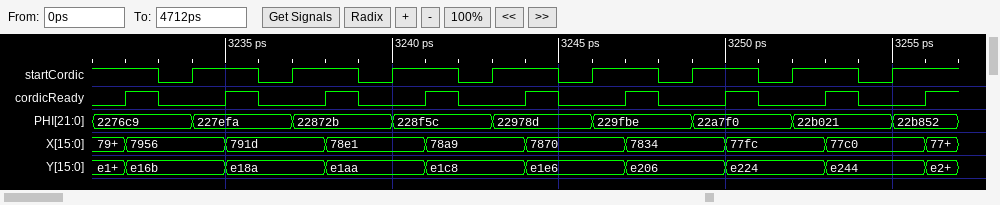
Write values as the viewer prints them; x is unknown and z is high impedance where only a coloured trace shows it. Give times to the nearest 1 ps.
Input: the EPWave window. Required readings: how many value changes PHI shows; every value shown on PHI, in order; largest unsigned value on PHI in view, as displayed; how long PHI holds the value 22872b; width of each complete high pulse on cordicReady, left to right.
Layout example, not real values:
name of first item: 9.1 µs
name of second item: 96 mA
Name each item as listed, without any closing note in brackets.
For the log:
how many value changes PHI shows: 8
every value shown on PHI, in order: 2276c9, 227efa, 22872b, 228f5c, 22978d, 229fbe, 22a7f0, 22b021, 22b852
largest unsigned value on PHI in view, as displayed: 22b852
how long PHI holds the value 22872b: 3 ps
width of each complete high pulse on cordicReady, left to right: 1 ps, 1 ps, 1 ps, 1 ps, 1 ps, 1 ps, 1 ps, 1 ps
